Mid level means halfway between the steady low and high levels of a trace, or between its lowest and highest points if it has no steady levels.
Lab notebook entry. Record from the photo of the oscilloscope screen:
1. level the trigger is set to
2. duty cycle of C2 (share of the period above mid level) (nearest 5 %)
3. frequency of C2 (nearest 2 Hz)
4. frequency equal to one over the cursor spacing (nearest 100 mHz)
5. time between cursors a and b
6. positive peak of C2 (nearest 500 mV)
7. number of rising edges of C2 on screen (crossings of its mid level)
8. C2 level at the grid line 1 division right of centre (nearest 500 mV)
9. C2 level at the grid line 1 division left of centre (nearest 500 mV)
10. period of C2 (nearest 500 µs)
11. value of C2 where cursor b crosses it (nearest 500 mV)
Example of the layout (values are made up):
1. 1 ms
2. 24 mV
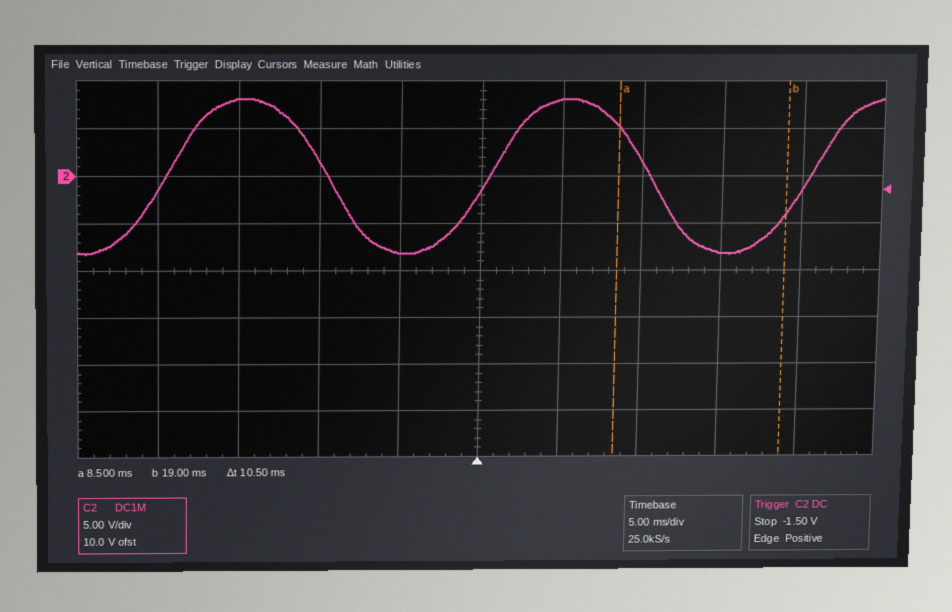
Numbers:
1. -1.50 V
2. 50 %
3. 50 Hz
4. 95.2 Hz
5. 10.5 ms
6. 8.0 V
7. 3
8. 8.0 V
9. -8.0 V
10. 20.0 ms
11. -4.0 V
